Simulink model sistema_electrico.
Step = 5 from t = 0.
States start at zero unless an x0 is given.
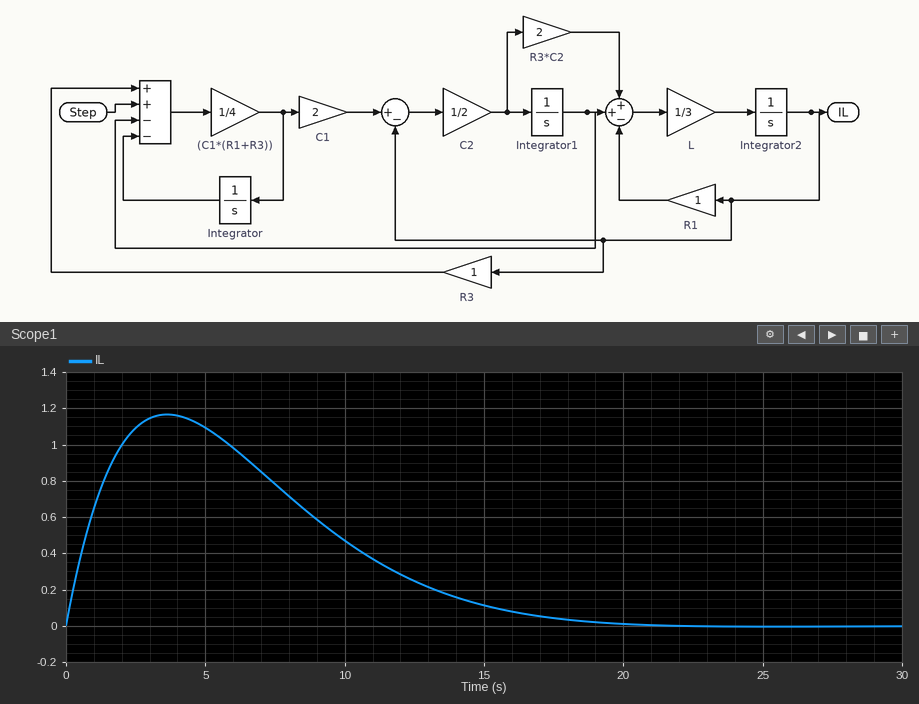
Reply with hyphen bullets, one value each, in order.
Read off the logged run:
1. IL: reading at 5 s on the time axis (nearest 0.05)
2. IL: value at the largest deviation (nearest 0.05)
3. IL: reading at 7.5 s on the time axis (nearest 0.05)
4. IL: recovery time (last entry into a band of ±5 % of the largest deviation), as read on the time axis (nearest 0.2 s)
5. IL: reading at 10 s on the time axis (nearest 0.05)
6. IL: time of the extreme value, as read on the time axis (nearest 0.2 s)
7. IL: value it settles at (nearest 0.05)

- 1.10
- 1.15
- 0.80
- 16.8 s
- 0.45
- 3.6 s
- 0.00
